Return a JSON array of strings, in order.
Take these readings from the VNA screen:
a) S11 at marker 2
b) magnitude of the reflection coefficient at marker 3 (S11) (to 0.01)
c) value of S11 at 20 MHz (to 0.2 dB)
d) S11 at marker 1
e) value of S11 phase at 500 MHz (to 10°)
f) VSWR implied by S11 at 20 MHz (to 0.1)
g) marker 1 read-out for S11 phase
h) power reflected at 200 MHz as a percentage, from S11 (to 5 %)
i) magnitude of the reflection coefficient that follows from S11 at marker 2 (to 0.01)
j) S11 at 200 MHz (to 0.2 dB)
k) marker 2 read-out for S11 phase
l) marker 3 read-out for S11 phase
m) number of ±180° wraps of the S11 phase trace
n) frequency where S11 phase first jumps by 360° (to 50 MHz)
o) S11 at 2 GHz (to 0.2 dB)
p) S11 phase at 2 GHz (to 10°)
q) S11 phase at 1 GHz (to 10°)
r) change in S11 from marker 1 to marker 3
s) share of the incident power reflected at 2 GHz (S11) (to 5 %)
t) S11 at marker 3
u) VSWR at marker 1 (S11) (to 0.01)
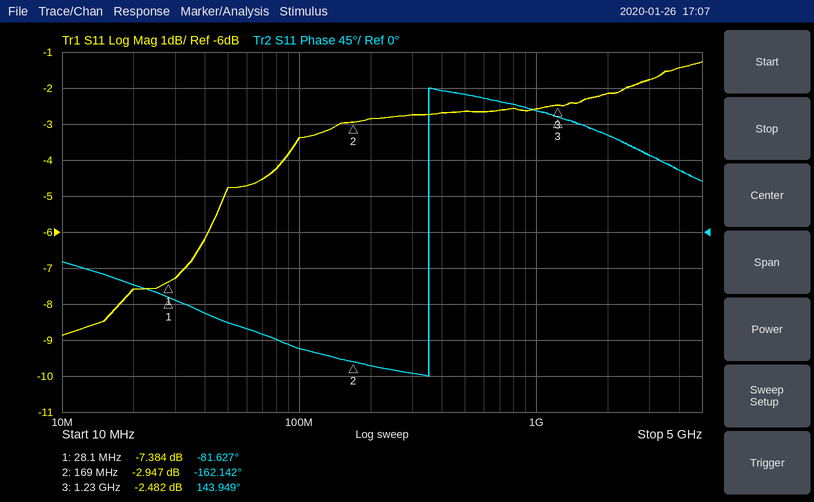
["-2.947 dB", "0.75", "-7.6 dB", "-7.384 dB", "170°", "2.4", "-81.627°", "50 %", "0.71", "-2.8 dB", "-162.142°", "143.949°", "1", "350 MHz", "-2.2 dB", "120°", "150°", "4.902 dB", "60 %", "-2.482 dB", "2.49"]
